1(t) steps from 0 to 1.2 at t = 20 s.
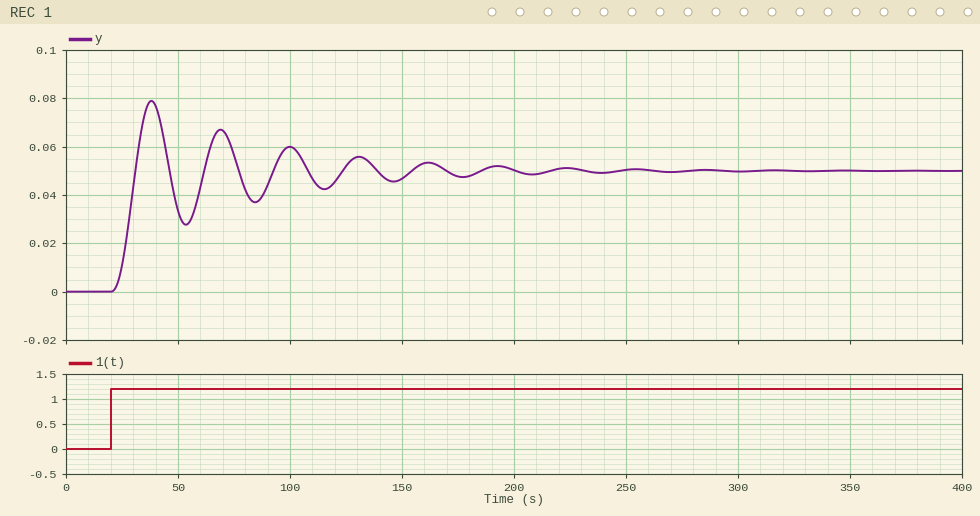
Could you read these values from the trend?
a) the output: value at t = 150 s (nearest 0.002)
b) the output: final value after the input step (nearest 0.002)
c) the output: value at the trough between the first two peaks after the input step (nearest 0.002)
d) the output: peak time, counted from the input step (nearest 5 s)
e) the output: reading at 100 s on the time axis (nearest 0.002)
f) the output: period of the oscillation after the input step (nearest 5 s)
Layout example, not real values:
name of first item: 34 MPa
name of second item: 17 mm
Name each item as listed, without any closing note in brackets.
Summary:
the output: value at t = 150 s: 0.046
the output: final value after the input step: 0.050
the output: value at the trough between the first two peaks after the input step: 0.028
the output: peak time, counted from the input step: 20 s
the output: reading at 100 s on the time axis: 0.060
the output: period of the oscillation after the input step: 30 s
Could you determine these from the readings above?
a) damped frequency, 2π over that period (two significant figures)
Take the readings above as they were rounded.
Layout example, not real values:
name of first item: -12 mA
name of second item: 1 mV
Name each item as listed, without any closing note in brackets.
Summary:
damped frequency, 2π over that period: 0.21 rad/s
